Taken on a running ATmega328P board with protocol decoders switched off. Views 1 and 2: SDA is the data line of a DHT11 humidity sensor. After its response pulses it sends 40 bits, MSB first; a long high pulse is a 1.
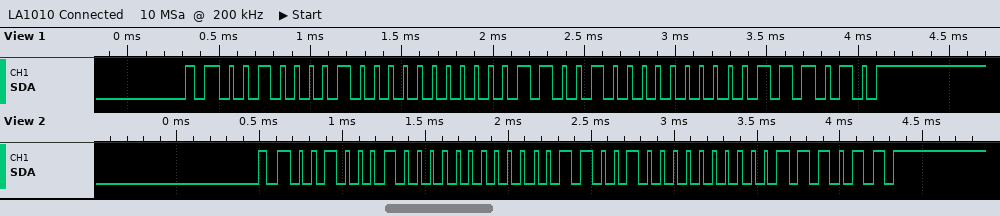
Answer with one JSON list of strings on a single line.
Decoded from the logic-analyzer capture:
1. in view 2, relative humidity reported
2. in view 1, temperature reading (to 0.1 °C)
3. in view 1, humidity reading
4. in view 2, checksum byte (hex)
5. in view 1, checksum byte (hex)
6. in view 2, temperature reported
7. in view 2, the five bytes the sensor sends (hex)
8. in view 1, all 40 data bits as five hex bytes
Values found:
["34 %", "25.0 °C", "33 %", "0x3B", "0x3A", "25.0 °C", "22 00 19 00 3B", "21 00 19 00 3A"]
